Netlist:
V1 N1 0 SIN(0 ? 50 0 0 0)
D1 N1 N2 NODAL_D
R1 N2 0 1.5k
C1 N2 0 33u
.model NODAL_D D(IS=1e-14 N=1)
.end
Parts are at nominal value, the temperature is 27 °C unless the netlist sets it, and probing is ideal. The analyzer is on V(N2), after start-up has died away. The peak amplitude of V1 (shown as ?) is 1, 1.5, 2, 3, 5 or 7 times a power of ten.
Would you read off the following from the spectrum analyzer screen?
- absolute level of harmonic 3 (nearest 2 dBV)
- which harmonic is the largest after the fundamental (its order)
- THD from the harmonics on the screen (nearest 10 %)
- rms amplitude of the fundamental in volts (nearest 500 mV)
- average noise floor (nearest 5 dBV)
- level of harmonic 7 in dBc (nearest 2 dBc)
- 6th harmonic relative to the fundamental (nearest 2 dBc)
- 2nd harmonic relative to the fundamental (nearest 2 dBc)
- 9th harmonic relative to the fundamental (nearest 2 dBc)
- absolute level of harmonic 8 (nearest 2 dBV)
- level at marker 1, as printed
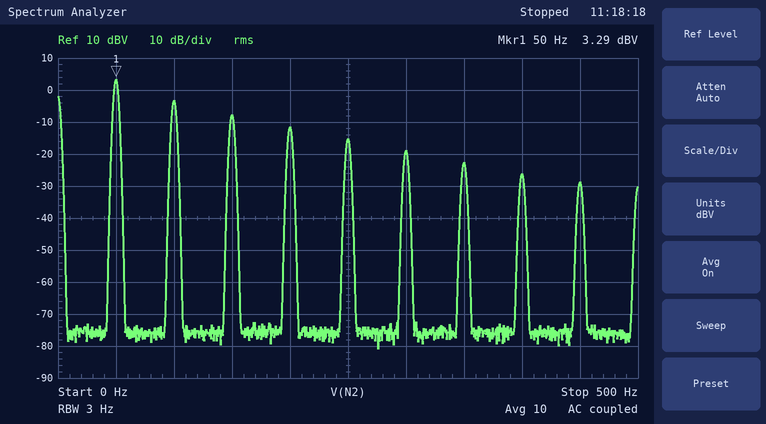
-8 dBV
2
60 %
1.5 V
-75 dBV
-26 dBc
-22 dBc
-6 dBc
-32 dBc
-26 dBV
3.29 dBV
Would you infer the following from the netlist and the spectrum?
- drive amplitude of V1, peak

20 V
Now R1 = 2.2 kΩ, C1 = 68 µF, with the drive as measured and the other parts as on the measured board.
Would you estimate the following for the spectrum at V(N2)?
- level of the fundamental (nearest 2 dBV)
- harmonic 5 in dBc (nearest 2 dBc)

-6 dBV
-16 dBc
